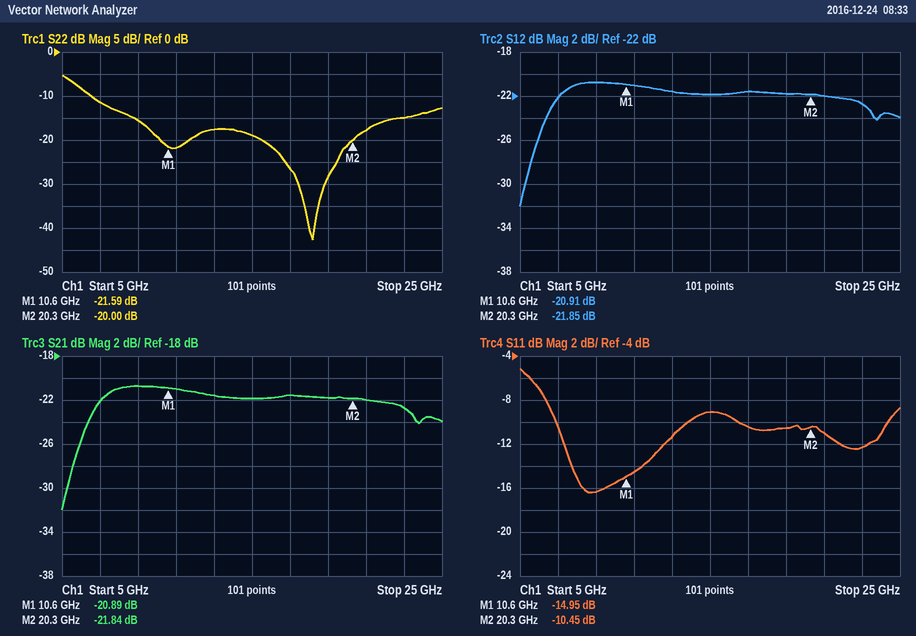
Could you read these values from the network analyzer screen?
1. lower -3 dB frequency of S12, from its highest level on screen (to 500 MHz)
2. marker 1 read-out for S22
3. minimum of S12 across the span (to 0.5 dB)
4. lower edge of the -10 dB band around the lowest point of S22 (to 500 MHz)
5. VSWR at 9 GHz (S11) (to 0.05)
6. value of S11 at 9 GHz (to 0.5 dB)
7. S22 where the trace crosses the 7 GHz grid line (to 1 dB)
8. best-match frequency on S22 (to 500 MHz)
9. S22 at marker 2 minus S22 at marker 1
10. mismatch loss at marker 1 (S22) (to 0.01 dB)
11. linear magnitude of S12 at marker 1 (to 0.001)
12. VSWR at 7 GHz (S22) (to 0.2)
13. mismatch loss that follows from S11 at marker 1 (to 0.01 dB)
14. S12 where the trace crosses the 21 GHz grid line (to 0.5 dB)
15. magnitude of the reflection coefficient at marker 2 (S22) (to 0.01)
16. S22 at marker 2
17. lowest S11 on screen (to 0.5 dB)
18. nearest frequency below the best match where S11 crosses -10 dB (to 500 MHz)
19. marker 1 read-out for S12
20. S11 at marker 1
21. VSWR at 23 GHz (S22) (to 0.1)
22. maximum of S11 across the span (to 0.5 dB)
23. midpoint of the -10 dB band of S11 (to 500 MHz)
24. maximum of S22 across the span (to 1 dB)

6.5 GHz
-21.59 dB
-32.0 dB
6.5 GHz
1.35
-16.5 dB
-11 dB
18.0 GHz
1.59 dB
0.03 dB
0.090
1.8
0.14 dB
-22.0 dB
0.10
-20.00 dB
-16.5 dB
7.0 GHz
-20.91 dB
-14.95 dB
1.4
-5.0 dB
10.5 GHz
-5 dB
